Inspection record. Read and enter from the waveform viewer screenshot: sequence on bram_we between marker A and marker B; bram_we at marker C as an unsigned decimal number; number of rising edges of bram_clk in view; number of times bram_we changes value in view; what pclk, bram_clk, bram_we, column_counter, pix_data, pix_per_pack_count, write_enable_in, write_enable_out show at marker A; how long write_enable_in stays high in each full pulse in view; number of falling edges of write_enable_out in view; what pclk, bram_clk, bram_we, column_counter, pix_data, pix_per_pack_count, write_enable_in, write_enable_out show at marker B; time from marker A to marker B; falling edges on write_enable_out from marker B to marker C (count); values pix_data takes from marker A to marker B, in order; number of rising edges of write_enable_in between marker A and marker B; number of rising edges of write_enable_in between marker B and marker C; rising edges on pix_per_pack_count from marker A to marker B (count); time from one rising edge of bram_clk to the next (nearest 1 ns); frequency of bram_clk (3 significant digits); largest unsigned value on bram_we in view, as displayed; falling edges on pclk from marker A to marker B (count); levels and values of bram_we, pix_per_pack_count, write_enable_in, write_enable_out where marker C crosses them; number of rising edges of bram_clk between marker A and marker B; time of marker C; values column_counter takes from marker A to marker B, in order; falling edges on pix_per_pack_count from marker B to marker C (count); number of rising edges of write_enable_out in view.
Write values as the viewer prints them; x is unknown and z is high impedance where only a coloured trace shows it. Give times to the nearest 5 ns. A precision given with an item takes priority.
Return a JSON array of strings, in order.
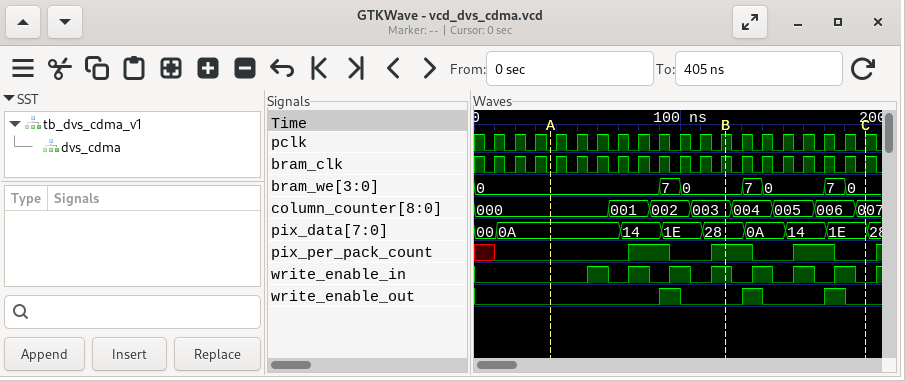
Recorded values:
["0, 7, 0", "0", "19", "6", "pclk=0, bram_clk=0, bram_we=0, column_counter=000, pix_data=0A, pix_per_pack_count=0, write_enable_in=0, write_enable_out=0", "10 ns, 10 ns, 10 ns, 10 ns, 10 ns, 10 ns, 10 ns", "3", "pclk=1, bram_clk=1, bram_we=0, column_counter=003, pix_data=28, pix_per_pack_count=1, write_enable_in=1, write_enable_out=0", "85 ns", "2", "0A, 14, 1E, 28", "4", "3", "2", "10 ns", "100 MHz", "7", "8", "bram_we=0, pix_per_pack_count=0, write_enable_in=0, write_enable_out=0", "9", "190 ns", "000, 001, 002, 003", "2", "3"]
